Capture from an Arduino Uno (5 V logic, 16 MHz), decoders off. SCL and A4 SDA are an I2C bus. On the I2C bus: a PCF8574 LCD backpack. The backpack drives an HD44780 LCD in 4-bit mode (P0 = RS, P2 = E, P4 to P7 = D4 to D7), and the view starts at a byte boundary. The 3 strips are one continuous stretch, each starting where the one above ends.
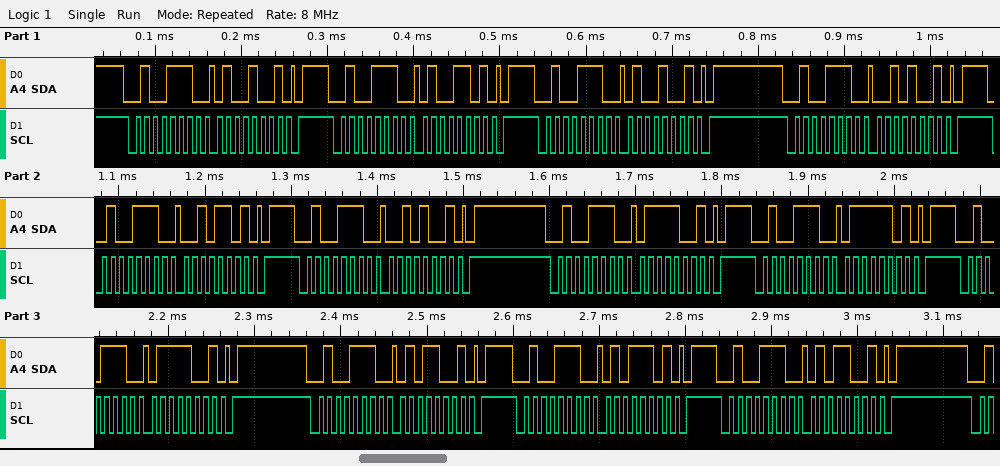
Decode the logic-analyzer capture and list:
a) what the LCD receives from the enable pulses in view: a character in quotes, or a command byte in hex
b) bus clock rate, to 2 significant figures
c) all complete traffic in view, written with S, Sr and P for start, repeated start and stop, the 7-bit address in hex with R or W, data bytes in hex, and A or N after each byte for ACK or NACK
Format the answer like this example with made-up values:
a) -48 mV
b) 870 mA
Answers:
a) 'B' 'u'
b) 100 kHz
c) S 27W A 49 A P S 27W A 4D A P S 27W A 49 A P S 27W A 29 A P S 27W A 2D A P S 27W A 29 A P S 27W A 79 A P S 27W A 7D A P S 27W A 79 A P S 27W A 59 A P S 27W A 5D A P S 27W A 59 A P
